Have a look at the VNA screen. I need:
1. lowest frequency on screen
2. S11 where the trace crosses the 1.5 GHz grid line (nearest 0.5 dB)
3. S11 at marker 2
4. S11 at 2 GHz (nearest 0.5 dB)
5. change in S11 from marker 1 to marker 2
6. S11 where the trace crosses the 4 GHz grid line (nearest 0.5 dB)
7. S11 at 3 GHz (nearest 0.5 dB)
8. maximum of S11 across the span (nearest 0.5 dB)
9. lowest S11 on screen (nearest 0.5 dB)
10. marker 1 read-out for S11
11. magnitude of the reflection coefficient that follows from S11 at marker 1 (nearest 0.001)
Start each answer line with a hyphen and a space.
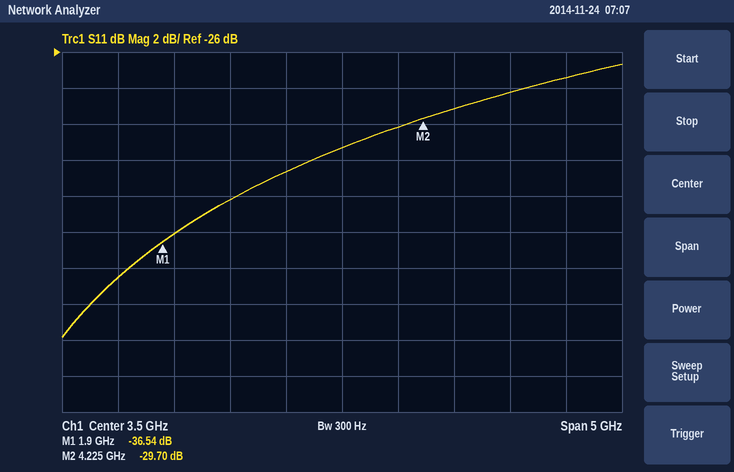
- 1 GHz
- -38.5 dB
- -29.70 dB
- -36.0 dB
- 6.84 dB
- -30.0 dB
- -32.5 dB
- -26.5 dB
- -42.0 dB
- -36.54 dB
- 0.015
